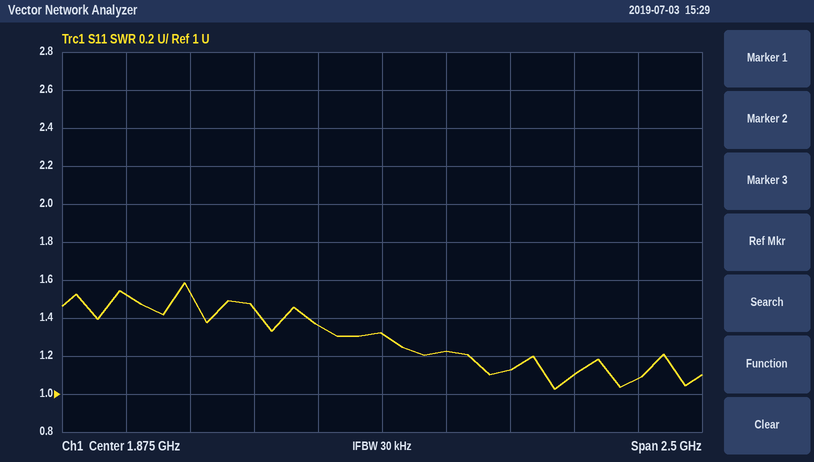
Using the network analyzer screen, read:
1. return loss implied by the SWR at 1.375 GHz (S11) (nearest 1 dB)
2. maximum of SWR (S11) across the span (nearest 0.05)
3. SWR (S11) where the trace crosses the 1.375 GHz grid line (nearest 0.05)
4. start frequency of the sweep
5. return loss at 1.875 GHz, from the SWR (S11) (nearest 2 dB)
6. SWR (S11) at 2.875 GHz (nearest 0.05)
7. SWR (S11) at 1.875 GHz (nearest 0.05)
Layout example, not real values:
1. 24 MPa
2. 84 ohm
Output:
1. 15 dB
2. 1.60
3. 1.45
4. 625 MHz
5. 18 dB
6. 1.10
7. 1.30
